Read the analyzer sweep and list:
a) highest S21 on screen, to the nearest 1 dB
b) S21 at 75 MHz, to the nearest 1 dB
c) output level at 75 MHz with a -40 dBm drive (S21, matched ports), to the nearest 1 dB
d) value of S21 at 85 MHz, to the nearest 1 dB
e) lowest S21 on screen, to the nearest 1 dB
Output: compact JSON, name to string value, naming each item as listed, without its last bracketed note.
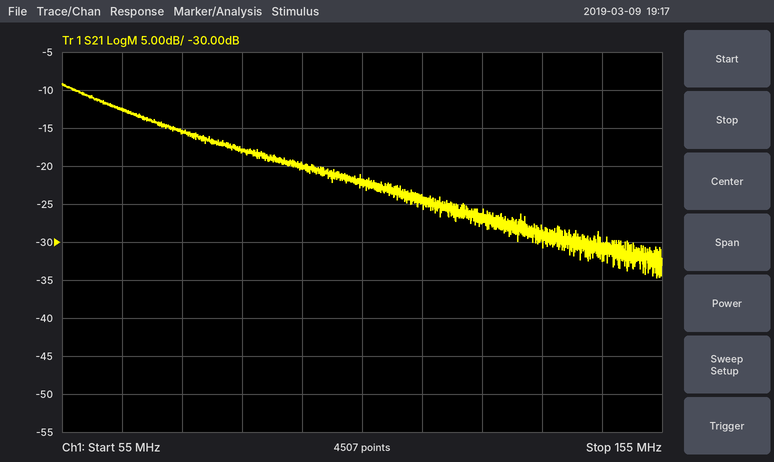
{"highest S21 on screen, to the nearest 1 dB": "-9 dB", "S21 at 75 MHz, to the nearest 1 dB": "-15 dB", "output level at 75 MHz with a -40 dBm drive (S21, matched ports), to the nearest 1 dB": "-55 dBm", "value of S21 at 85 MHz, to the nearest 1 dB": "-18 dB", "lowest S21 on screen, to the nearest 1 dB": "-35 dB"}
